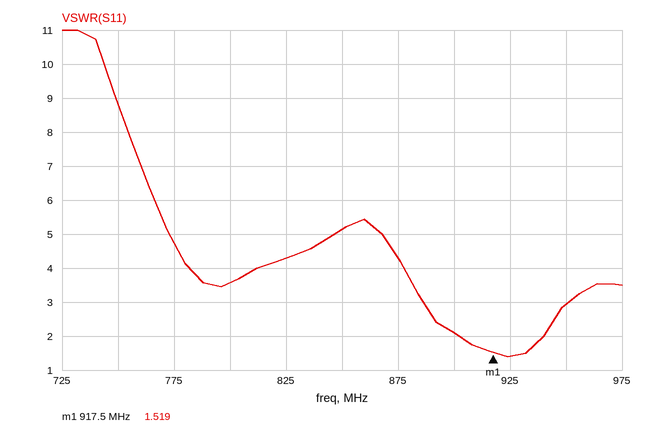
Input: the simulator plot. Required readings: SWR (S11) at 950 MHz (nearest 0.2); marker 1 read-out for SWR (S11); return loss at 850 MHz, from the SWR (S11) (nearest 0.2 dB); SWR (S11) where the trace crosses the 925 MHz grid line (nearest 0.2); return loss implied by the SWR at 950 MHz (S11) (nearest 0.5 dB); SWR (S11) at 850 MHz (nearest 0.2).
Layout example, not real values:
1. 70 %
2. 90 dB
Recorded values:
1. 3.0
2. 1.519
3. 3.4 dB
4. 1.4
5. 6.0 dB
6. 5.2
